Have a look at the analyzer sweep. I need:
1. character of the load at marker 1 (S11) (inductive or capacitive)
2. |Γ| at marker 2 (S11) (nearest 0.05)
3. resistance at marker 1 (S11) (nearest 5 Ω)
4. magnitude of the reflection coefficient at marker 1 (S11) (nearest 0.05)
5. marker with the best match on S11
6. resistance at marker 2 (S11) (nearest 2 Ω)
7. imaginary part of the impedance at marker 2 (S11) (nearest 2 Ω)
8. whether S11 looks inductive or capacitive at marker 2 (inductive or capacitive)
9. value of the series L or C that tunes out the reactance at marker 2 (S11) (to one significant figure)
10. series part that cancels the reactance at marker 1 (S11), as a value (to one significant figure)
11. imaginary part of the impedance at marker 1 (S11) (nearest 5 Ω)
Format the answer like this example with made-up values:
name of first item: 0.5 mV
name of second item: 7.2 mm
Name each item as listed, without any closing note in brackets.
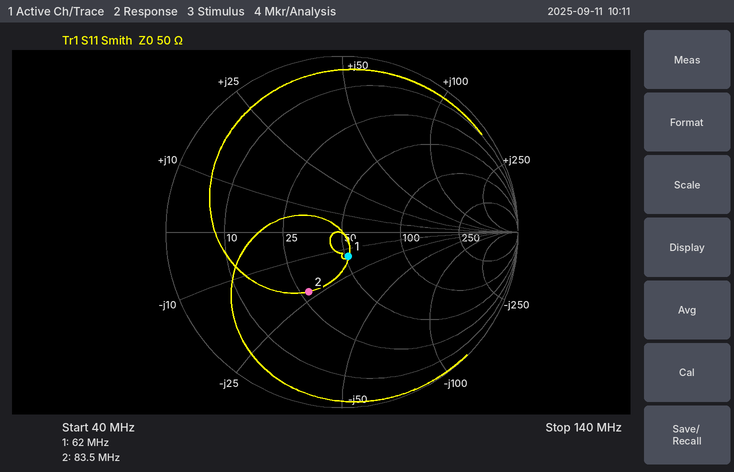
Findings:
character of the load at marker 1 (S11): capacitive
|Γ| at marker 2 (S11): 0.40
resistance at marker 1 (S11): 50 Ω
magnitude of the reflection coefficient at marker 1 (S11): 0.15
marker with the best match on S11: marker 1
resistance at marker 2 (S11): 28 Ω
imaginary part of the impedance at marker 2 (S11): -22 Ω
whether S11 looks inductive or capacitive at marker 2: capacitive
value of the series L or C that tunes out the reactance at marker 2 (S11): 40 nH
series part that cancels the reactance at marker 1 (S11), as a value: 40 nH
imaginary part of the impedance at marker 1 (S11): -15 Ω
